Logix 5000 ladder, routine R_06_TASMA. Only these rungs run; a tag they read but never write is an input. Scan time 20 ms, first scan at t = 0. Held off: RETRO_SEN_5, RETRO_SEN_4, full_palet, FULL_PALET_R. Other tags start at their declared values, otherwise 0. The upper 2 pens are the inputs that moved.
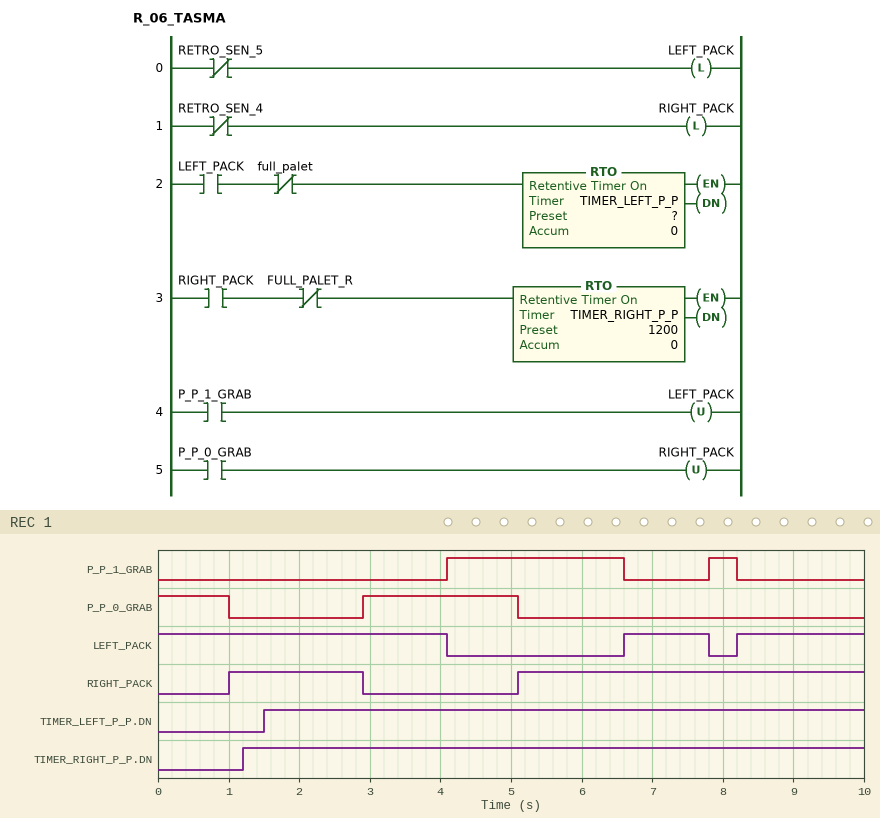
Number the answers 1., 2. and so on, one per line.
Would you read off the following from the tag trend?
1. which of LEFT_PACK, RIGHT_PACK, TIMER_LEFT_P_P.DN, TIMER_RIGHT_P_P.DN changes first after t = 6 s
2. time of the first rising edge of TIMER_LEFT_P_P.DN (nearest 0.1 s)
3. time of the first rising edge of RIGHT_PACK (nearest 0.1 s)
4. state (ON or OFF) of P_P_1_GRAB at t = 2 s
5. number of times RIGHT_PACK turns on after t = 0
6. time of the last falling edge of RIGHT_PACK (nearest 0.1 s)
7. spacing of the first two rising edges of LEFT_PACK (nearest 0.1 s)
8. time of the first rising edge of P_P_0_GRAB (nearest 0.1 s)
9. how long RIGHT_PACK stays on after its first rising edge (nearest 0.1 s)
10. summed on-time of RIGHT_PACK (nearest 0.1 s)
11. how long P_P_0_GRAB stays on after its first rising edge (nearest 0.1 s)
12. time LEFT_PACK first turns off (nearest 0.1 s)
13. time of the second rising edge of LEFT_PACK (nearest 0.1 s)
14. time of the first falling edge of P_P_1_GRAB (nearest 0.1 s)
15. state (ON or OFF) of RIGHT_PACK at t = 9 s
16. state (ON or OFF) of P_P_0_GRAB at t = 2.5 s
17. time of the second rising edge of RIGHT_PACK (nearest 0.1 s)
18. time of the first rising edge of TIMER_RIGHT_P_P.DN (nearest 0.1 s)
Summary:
1. LEFT_PACK
2. 1.5 s
3. 1.0 s
4. OFF
5. 2
6. 2.9 s
7. 1.6 s
8. 2.9 s
9. 1.9 s
10. 6.8 s
11. 2.2 s
12. 4.1 s
13. 8.2 s
14. 6.6 s
15. ON
16. OFF
17. 5.1 s
18. 1.2 s
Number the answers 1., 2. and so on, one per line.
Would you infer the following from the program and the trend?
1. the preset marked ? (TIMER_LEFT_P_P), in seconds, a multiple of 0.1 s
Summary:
1. 1.5 s
